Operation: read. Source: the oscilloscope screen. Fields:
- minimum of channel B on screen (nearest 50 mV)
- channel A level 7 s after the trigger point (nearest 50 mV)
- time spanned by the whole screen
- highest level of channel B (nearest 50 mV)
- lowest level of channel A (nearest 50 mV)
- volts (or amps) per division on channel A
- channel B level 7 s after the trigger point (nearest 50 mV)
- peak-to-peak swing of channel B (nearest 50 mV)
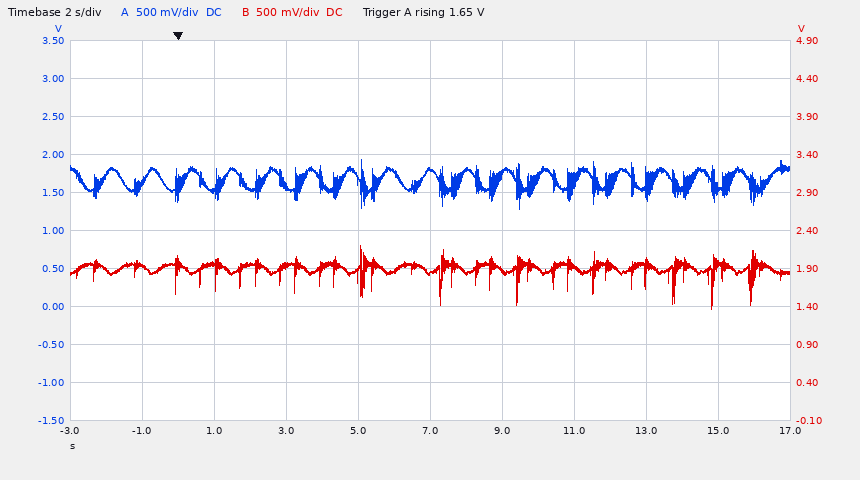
1.35 V
1.80 V
20 s
2.20 V
1.30 V
500 mV
1.85 V
850 mV
